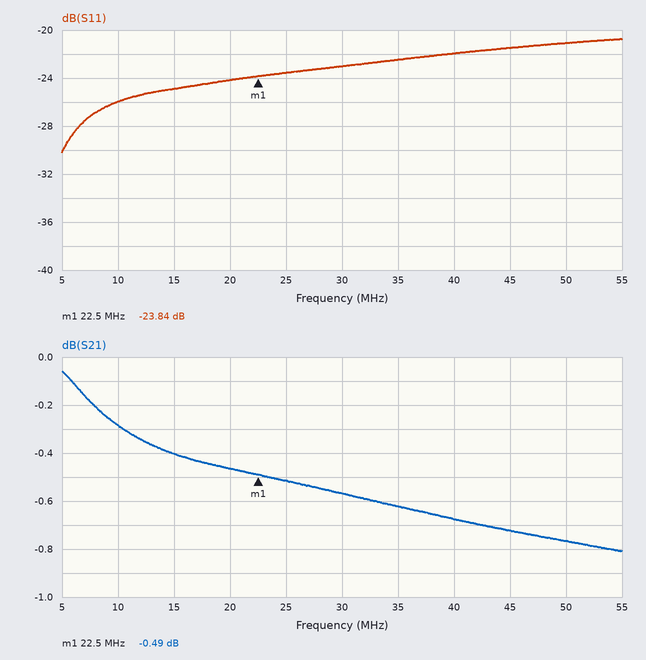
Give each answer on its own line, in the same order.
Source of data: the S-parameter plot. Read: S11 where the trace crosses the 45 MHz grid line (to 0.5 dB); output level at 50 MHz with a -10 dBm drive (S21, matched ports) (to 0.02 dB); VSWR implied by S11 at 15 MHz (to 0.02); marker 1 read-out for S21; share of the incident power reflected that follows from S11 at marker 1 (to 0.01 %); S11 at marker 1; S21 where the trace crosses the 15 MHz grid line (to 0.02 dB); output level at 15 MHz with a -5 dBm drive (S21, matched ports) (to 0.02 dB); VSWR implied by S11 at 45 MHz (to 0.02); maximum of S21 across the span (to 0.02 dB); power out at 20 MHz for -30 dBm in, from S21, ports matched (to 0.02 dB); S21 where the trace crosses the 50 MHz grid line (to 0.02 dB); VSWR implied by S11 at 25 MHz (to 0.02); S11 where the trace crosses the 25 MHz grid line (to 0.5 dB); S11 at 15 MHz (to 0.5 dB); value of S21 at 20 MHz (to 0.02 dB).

-21.5 dB
-10.76 dBm
1.12
-0.49 dB
0.41 %
-23.84 dB
-0.40 dB
-5.40 dBm
1.18
-0.06 dB
-30.46 dBm
-0.76 dB
1.14
-23.5 dB
-25.0 dB
-0.46 dB
